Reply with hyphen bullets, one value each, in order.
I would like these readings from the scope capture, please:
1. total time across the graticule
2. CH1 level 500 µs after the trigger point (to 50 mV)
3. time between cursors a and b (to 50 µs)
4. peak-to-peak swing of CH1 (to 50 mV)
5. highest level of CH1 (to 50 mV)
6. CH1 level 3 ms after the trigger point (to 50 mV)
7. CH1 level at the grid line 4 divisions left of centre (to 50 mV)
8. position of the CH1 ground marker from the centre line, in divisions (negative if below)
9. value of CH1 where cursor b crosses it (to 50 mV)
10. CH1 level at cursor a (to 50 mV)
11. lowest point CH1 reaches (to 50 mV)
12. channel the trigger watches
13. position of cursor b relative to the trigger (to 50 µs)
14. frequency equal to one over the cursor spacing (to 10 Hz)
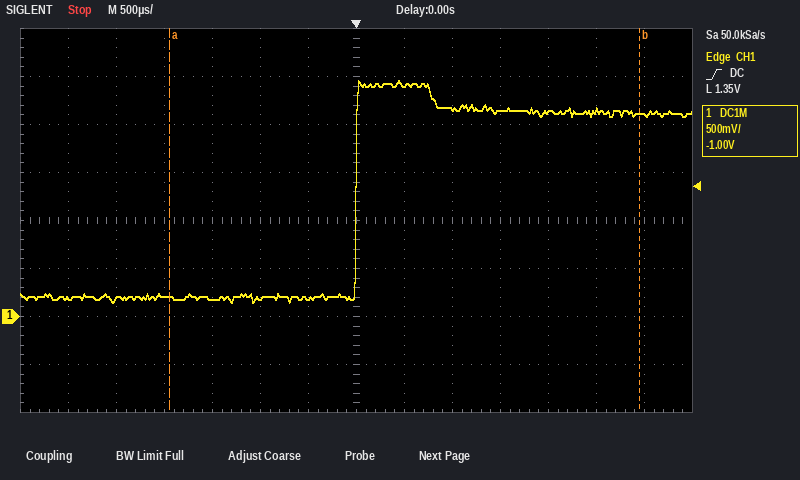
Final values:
- 7 ms
- 2.40 V
- 4.90 ms
- 2.30 V
- 2.45 V
- 2.10 V
- 200 mV
- -2.0 div
- 2.10 V
- 200 mV
- 150 mV
- CH1
- +2.95 ms
- 200 Hz
